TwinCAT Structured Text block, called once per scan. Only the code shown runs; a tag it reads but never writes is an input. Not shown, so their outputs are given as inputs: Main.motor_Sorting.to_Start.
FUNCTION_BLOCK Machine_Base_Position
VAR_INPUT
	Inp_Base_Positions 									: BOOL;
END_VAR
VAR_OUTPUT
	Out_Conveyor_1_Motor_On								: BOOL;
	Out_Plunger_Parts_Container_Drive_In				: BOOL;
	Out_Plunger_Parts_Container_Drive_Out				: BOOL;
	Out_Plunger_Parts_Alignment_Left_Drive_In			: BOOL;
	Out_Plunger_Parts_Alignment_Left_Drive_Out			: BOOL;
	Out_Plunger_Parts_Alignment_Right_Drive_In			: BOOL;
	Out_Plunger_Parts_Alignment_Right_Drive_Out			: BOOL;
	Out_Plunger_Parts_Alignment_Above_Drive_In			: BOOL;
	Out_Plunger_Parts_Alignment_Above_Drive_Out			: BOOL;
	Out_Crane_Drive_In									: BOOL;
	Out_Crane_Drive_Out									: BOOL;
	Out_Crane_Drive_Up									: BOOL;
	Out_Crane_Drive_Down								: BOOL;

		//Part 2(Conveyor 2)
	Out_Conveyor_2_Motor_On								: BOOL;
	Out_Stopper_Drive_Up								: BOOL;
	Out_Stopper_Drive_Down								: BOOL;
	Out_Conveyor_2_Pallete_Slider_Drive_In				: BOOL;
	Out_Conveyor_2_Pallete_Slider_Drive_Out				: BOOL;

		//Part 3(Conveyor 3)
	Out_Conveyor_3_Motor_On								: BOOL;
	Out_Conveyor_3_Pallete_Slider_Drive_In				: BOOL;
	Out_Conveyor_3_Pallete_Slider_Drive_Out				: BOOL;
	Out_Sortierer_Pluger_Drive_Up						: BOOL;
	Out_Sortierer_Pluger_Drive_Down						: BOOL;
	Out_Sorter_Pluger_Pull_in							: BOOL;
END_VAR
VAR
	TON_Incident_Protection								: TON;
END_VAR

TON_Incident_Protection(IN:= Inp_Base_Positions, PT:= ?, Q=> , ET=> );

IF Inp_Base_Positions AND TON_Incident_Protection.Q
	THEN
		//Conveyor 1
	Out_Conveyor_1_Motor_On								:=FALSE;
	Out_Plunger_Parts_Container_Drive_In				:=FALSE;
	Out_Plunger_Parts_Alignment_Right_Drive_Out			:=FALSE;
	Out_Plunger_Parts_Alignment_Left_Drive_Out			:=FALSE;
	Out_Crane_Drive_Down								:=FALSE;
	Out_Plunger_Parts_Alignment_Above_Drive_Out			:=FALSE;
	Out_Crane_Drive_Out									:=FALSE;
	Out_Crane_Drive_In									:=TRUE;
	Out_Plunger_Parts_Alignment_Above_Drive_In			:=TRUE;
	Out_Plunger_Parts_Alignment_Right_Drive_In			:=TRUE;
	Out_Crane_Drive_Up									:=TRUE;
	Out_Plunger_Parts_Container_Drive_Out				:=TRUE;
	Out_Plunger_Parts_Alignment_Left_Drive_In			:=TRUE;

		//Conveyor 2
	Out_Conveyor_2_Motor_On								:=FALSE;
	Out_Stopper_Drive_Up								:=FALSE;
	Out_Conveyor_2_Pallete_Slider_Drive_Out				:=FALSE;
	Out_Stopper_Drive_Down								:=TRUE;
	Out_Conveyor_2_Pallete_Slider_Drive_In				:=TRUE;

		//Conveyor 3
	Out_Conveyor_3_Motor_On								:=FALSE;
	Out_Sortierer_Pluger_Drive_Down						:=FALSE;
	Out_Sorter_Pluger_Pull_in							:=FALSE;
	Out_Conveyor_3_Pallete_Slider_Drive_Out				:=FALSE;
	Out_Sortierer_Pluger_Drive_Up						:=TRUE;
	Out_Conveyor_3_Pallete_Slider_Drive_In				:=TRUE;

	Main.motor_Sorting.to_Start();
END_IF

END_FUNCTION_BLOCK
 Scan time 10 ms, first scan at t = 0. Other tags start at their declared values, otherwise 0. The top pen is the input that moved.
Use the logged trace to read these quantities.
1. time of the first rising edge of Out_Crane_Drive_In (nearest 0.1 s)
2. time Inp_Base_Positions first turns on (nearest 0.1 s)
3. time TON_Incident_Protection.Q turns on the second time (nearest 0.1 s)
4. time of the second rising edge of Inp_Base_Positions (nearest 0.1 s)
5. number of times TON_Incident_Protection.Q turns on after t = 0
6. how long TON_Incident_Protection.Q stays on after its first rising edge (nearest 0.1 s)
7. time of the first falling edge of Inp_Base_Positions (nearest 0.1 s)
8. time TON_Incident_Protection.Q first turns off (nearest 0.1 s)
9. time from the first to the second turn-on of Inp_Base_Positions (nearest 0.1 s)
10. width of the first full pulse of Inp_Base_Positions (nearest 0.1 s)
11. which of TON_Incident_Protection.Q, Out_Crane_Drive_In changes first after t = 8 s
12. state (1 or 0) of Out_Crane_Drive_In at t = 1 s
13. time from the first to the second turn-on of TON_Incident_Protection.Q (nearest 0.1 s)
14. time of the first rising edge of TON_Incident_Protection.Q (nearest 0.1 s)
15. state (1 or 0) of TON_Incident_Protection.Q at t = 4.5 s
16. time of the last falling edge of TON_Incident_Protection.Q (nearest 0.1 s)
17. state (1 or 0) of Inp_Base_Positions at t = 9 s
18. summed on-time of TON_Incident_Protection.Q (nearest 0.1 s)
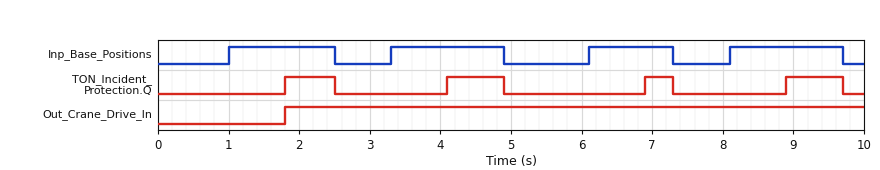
1.8 s
1.0 s
4.1 s
3.3 s
4
0.7 s
2.5 s
2.5 s
2.3 s
1.5 s
TON_Incident_Protection.Q
0
2.3 s
1.8 s
1
9.7 s
1
2.7 s
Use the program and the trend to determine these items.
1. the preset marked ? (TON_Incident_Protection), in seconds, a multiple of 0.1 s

0.8 s
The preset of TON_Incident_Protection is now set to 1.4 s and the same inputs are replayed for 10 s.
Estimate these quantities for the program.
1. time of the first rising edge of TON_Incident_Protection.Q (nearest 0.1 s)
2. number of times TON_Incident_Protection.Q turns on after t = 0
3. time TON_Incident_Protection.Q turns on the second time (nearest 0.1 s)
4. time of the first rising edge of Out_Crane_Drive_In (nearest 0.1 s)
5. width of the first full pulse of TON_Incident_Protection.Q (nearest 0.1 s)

2.4 s
3
4.7 s
2.4 s
0.1 s
